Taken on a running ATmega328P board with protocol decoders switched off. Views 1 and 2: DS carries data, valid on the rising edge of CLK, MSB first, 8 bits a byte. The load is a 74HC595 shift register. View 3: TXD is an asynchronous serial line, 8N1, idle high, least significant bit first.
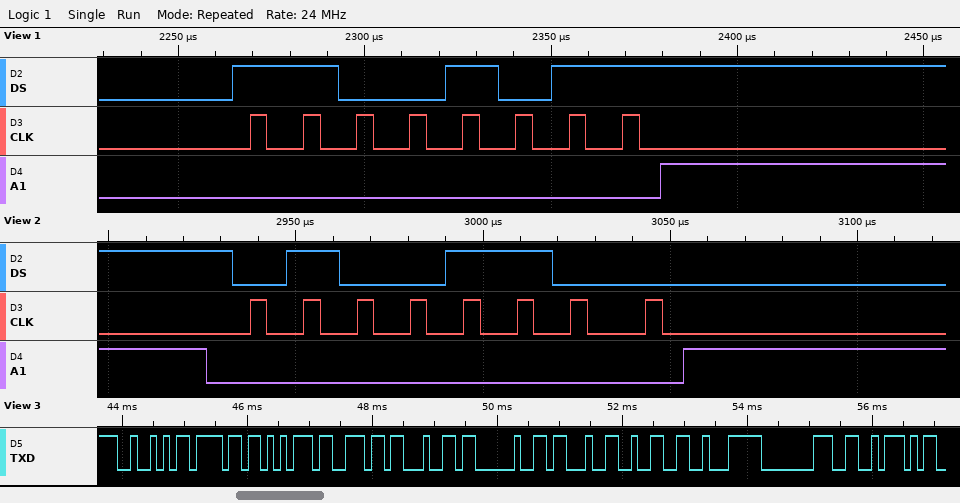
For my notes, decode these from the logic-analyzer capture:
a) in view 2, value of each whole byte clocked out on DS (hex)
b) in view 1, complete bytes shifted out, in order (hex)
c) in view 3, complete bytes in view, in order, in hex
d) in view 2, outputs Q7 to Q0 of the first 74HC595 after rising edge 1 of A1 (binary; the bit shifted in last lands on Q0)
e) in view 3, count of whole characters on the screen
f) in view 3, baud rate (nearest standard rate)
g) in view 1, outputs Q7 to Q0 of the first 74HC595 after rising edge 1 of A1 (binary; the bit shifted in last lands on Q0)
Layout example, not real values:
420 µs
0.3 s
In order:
4C
CB
52 6F 75 6E 64 20 23 32 E2 80 A6
01001100
11
9600 baud
11001011
